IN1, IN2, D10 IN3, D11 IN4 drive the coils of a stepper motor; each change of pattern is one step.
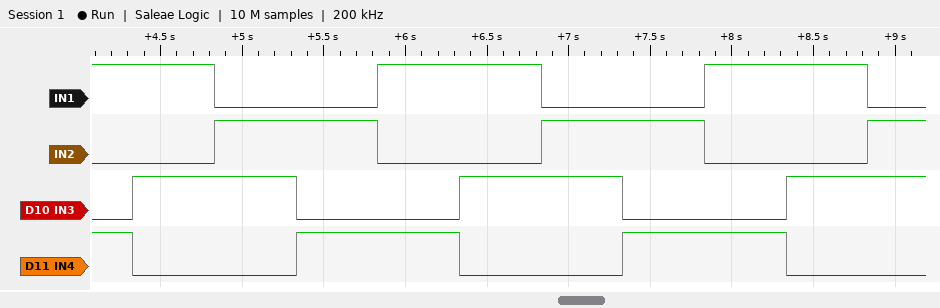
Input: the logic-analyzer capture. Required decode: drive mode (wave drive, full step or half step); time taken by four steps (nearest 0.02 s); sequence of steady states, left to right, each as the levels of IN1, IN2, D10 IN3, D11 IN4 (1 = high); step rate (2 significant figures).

full step
2.00 s
1001 1010 0110 0101 1001 1010 0110 0101 1001 1010 0110
2.0 steps/s
